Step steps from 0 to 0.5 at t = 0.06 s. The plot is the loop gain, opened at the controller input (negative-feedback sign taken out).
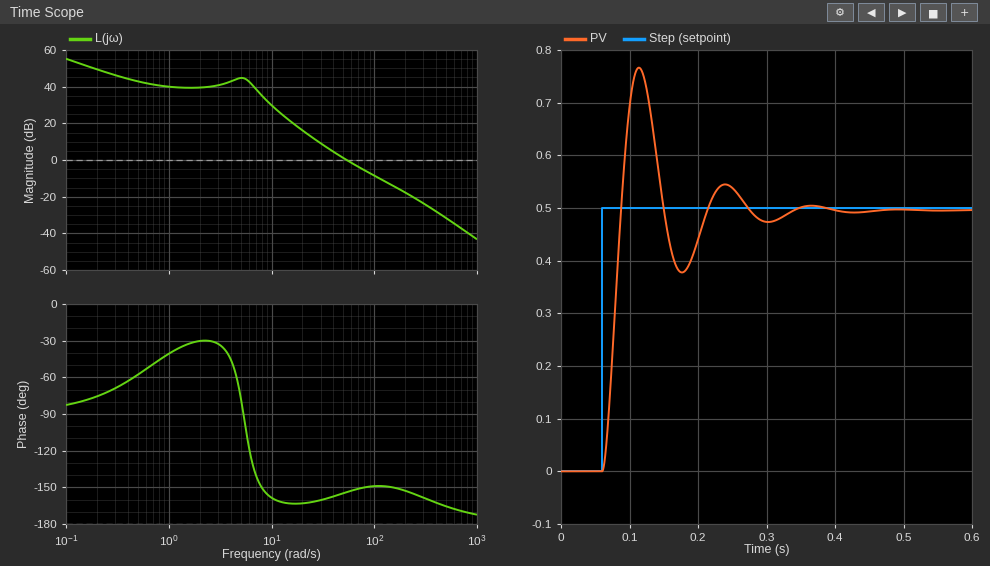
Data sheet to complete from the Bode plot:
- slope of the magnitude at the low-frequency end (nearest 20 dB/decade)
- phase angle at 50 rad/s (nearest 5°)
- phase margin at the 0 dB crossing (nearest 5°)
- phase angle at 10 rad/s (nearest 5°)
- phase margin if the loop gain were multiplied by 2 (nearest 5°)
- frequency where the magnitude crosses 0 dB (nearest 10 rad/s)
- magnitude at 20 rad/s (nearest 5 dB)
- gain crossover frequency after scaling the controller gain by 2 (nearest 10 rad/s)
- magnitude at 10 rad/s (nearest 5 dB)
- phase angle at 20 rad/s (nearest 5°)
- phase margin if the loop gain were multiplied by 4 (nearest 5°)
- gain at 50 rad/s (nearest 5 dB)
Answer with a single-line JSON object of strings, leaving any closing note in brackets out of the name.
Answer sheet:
{"slope of the magnitude at the low-frequency end": "-20 dB/decade", "phase angle at 50 rad/s": "-155°", "phase margin at the 0 dB crossing": "25°", "phase angle at 10 rad/s": "-160°", "phase margin if the loop gain were multiplied by 2": "30°", "frequency where the magnitude crosses 0 dB": "50 rad/s", "magnitude at 20 rad/s": "15 dB", "gain crossover frequency after scaling the controller gain by 2": "80 rad/s", "magnitude at 10 rad/s": "30 dB", "phase angle at 20 rad/s": "-165°", "phase margin if the loop gain were multiplied by 4": "30°", "gain at 50 rad/s": "0 dB"}
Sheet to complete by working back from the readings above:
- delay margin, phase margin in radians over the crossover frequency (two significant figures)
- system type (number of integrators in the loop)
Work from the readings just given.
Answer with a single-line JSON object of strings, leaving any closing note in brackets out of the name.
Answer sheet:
{"delay margin, phase margin in radians over the crossover frequency": "0.0087 s", "system type": "1"}
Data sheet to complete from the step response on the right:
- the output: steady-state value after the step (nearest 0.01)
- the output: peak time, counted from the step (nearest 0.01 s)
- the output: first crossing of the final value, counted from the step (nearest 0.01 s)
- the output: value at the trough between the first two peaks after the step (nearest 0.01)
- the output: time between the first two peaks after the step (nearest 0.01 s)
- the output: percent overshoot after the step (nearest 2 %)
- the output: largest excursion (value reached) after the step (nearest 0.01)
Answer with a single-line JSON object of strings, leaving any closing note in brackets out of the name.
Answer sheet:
{"the output: steady-state value after the step": "0.50", "the output: peak time, counted from the step": "0.05 s", "the output: first crossing of the final value, counted from the step": "0.03 s", "the output: value at the trough between the first two peaks after the step": "0.38", "the output: time between the first two peaks after the step": "0.13 s", "the output: percent overshoot after the step": "54 %", "the output: largest excursion (value reached) after the step": "0.77"}
